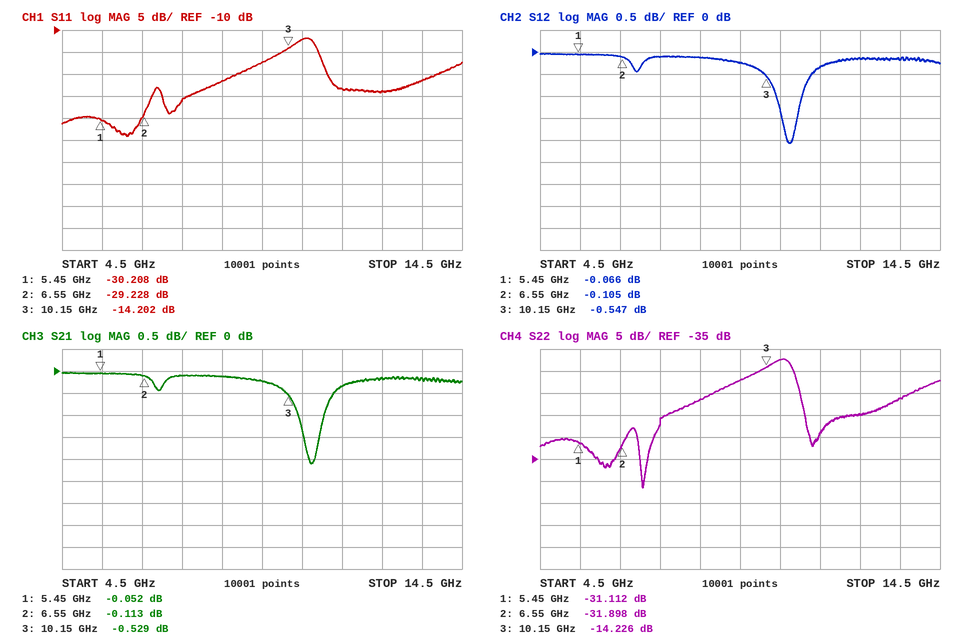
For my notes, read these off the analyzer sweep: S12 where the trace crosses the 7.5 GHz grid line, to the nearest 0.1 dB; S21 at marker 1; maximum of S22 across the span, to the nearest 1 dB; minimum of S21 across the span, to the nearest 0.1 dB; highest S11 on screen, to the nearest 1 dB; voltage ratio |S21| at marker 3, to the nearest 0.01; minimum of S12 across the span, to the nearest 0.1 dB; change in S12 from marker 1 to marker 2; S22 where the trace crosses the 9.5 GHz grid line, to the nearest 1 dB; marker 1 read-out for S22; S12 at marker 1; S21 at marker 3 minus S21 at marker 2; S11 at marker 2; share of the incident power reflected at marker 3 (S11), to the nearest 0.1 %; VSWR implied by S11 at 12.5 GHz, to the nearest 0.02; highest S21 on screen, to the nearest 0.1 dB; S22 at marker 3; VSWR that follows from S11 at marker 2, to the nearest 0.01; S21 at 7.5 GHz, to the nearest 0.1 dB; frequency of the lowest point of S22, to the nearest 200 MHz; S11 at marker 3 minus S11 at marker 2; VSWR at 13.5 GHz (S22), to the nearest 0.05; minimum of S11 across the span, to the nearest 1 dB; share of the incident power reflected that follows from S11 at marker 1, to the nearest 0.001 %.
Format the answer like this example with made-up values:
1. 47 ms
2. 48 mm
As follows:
1. -0.1 dB
2. -0.052 dB
3. -12 dB
4. -2.1 dB
5. -12 dB
6. 0.94
7. -2.1 dB
8. -0.039 dB
9. -17 dB
10. -31.112 dB
11. -0.066 dB
12. -0.416 dB
13. -29.228 dB
14. 3.8 %
15. 1.14
16. 0.0 dB
17. -14.226 dB
18. 1.07
19. -0.1 dB
20. 7.0 GHz
21. 15.026 dB
22. 1.20
23. -34 dB
24. 0.095 %
